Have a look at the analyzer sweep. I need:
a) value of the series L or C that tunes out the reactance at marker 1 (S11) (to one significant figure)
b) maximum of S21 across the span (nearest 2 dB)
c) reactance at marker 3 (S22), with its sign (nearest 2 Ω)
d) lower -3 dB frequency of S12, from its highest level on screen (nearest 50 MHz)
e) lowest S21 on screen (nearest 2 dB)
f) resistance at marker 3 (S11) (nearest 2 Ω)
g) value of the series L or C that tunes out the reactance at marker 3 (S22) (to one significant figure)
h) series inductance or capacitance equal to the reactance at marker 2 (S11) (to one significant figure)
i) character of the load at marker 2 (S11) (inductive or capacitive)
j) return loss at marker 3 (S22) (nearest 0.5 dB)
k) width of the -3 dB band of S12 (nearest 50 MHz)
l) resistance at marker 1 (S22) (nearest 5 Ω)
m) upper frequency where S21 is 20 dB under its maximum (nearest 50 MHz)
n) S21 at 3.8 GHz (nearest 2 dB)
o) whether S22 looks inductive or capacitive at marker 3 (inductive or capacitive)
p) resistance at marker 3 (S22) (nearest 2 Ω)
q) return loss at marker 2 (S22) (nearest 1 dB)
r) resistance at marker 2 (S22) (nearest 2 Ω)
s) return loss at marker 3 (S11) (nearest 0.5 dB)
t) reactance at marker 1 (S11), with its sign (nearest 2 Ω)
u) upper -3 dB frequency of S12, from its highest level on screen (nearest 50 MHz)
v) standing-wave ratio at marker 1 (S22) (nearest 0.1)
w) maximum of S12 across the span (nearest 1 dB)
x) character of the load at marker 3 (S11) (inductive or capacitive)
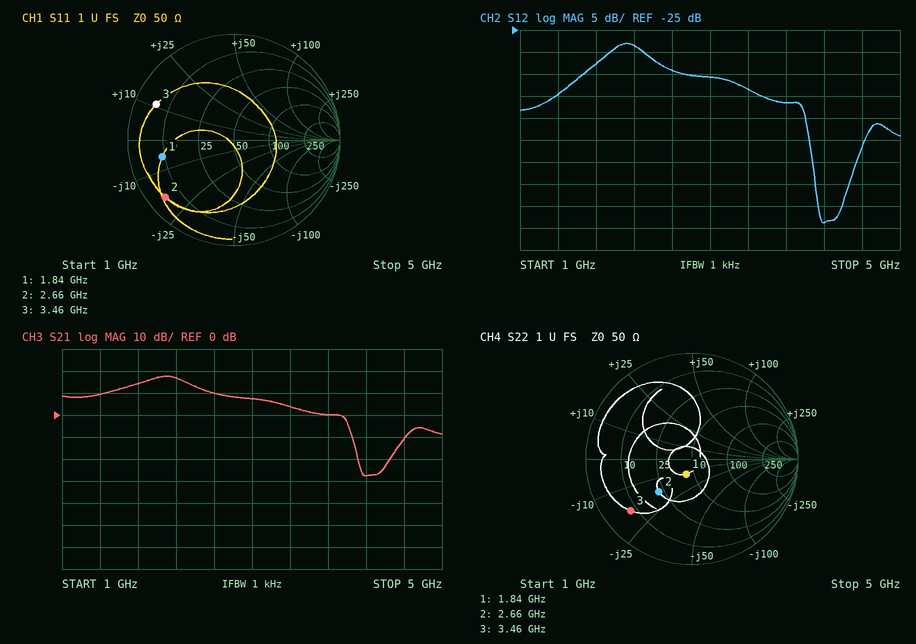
500 pH
18 dB
-18 Ω
1.90 GHz
-28 dB
6 Ω
800 pH
3 pF
capacitive
2.5 dB
450 MHz
45 Ω
4.00 GHz
0 dB
capacitive
8 Ω
7 dB
22 Ω
2.0 dB
-6 Ω
2.35 GHz
1.4
-28 dB
inductive
